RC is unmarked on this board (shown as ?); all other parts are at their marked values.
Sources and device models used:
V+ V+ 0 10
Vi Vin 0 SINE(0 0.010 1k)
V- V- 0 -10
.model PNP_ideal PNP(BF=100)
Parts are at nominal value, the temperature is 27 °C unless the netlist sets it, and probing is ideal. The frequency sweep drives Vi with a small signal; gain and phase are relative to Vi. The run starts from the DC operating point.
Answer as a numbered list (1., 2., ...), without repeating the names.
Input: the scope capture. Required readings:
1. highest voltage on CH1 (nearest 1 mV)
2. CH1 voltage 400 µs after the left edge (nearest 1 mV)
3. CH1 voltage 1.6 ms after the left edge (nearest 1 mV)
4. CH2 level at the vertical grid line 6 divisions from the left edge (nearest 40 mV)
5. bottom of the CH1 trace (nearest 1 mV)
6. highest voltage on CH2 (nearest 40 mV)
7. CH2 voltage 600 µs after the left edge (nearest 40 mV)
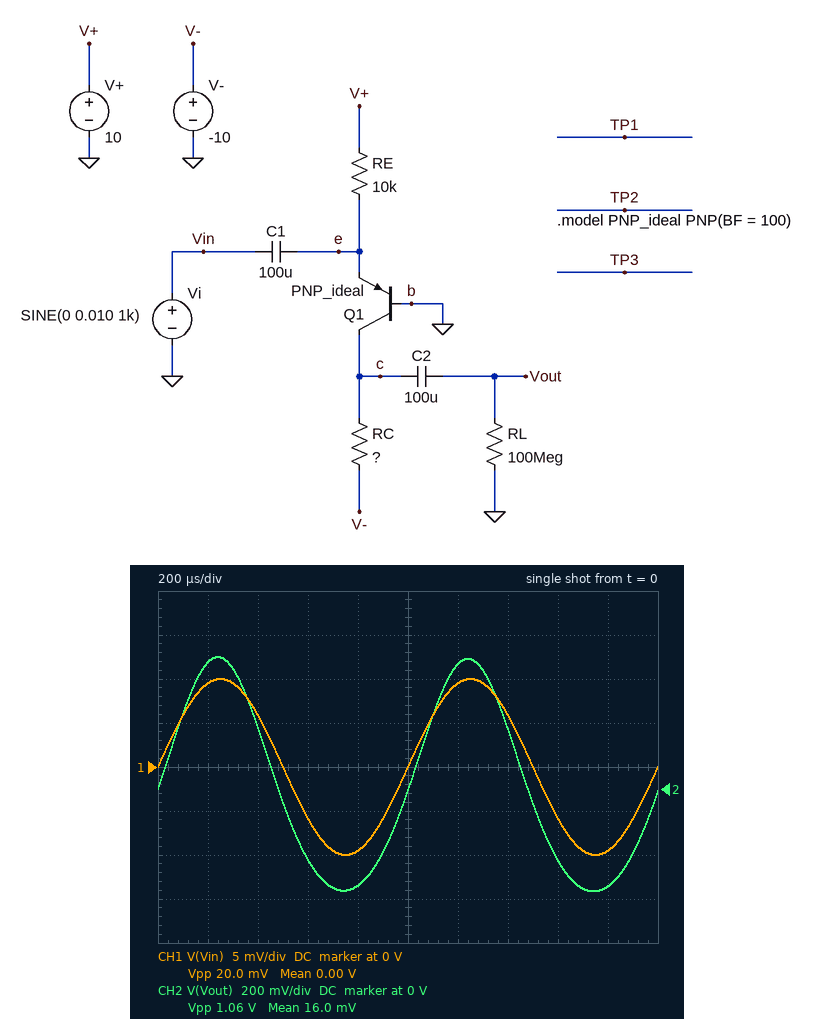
1. 10 mV
2. 6 mV
3. -6 mV
4. 560 mV
5. -10 mV
6. 600 mV
7. -320 mV
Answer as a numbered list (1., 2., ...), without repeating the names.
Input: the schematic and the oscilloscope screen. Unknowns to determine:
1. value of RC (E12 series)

1. 1.5 kΩ
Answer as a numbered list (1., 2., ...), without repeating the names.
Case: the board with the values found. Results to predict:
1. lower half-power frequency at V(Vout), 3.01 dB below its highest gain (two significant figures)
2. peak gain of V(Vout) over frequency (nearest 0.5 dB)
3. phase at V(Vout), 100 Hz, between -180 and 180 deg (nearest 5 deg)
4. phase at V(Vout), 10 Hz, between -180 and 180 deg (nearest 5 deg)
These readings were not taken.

1. 57 Hz
2. 34.5 dB
3. 30 deg
4. 80 deg
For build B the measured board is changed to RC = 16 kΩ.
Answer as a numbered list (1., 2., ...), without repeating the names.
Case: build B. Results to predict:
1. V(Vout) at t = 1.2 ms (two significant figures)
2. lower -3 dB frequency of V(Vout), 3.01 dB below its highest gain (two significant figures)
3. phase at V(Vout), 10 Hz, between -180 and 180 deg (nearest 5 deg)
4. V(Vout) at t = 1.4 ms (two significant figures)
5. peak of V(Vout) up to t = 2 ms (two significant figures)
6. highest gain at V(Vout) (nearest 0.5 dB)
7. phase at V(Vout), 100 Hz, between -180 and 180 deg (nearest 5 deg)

1. 18 mV
2. 36 Hz
3. 75 deg
4. 11 mV
5. 19 mV
6. 7.5 dB
7. 20 deg
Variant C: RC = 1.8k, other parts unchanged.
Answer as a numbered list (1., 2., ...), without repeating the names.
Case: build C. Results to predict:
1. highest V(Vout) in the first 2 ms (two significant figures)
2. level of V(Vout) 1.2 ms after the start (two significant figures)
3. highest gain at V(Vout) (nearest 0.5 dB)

1. 720 mV
2. 680 mV
3. 36.0 dB
